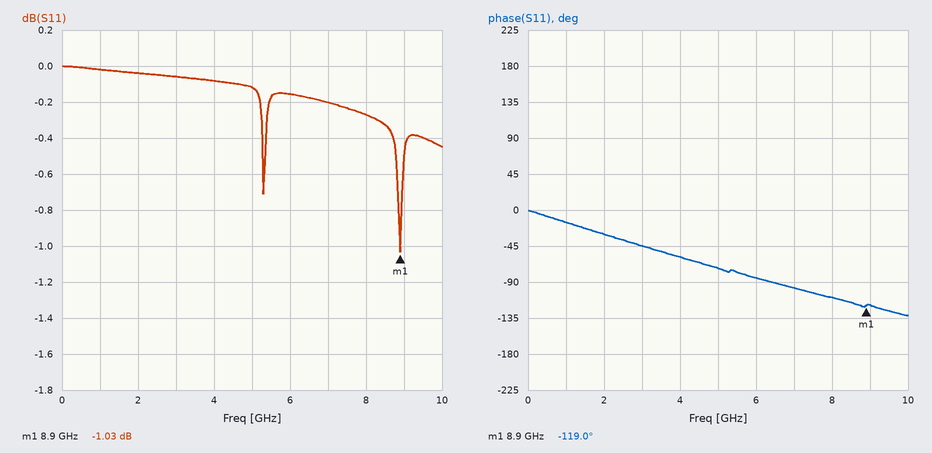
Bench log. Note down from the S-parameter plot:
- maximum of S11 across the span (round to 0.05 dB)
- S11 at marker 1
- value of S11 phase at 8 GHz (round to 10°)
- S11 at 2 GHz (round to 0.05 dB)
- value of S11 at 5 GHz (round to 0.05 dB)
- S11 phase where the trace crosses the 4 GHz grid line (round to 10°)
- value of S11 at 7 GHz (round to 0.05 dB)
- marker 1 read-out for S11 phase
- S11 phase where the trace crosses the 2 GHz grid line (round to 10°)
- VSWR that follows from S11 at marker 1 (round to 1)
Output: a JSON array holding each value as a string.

["0.00 dB", "-1.03 dB", "-110°", "-0.05 dB", "-0.10 dB", "-60°", "-0.20 dB", "-119.0°", "-30°", "17"]
